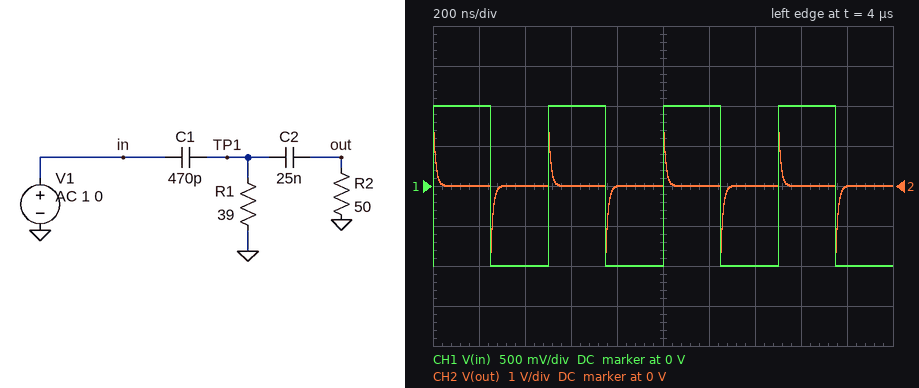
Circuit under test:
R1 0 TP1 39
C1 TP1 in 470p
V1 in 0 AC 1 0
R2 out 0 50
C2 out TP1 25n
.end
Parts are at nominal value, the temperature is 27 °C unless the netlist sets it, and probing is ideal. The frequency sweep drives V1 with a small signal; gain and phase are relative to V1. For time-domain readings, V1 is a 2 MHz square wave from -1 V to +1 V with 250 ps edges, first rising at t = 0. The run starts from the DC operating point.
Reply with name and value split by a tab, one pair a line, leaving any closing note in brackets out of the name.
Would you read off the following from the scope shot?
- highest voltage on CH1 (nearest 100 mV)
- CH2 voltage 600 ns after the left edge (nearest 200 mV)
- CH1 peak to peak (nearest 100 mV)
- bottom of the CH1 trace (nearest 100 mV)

highest voltage on CH1	1.0 V
CH2 voltage 600 ns after the left edge	0 V
CH1 peak to peak	2.0 V
bottom of the CH1 trace	-1.0 V
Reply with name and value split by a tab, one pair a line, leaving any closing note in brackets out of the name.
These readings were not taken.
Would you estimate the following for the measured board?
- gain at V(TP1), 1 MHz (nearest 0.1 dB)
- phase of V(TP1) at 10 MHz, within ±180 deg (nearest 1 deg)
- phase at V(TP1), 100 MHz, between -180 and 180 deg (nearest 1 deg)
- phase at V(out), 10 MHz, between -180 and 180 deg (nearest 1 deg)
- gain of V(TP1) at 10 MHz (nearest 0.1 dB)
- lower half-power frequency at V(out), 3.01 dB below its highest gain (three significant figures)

gain at V(TP1), 1 MHz	-23.8 dB
phase of V(TP1) at 10 MHz, within ±180 deg	57 deg
phase at V(TP1), 100 MHz, between -180 and 180 deg	9 deg
phase at V(out), 10 MHz, between -180 and 180 deg	58 deg
gain of V(TP1) at 10 MHz	-5.3 dB
lower half-power frequency at V(out), 3.01 dB below its highest gain	15.5 MHz
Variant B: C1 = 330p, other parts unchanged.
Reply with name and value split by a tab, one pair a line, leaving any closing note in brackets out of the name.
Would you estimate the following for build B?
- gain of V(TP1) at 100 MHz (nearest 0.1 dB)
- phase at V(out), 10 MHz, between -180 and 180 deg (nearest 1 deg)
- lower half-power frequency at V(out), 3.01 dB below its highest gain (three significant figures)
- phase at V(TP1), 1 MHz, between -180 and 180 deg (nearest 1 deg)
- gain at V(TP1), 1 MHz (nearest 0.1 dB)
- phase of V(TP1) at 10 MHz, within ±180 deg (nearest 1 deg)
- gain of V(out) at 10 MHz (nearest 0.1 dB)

gain of V(TP1) at 100 MHz	-0.2 dB
phase at V(out), 10 MHz, between -180 and 180 deg	66 deg
lower half-power frequency at V(out), 3.01 dB below its highest gain	22.1 MHz
phase at V(TP1), 1 MHz, between -180 and 180 deg	84 deg
gain at V(TP1), 1 MHz	-26.8 dB
phase of V(TP1) at 10 MHz, within ±180 deg	65 deg
gain of V(out) at 10 MHz	-7.7 dB
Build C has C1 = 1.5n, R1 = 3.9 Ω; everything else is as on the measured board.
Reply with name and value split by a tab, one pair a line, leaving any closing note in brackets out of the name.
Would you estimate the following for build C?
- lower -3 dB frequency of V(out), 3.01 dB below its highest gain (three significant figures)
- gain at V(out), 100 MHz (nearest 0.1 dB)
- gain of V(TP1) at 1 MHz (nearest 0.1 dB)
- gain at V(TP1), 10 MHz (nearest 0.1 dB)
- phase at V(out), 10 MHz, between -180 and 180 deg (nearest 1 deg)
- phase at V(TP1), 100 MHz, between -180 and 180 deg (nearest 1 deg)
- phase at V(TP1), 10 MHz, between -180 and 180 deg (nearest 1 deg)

lower -3 dB frequency of V(out), 3.01 dB below its highest gain	29.3 MHz
gain at V(out), 100 MHz	-0.4 dB
gain of V(TP1) at 1 MHz	-29.3 dB
gain at V(TP1), 10 MHz	-9.8 dB
phase at V(out), 10 MHz, between -180 and 180 deg	72 deg
phase at V(TP1), 100 MHz, between -180 and 180 deg	16 deg
phase at V(TP1), 10 MHz, between -180 and 180 deg	71 deg
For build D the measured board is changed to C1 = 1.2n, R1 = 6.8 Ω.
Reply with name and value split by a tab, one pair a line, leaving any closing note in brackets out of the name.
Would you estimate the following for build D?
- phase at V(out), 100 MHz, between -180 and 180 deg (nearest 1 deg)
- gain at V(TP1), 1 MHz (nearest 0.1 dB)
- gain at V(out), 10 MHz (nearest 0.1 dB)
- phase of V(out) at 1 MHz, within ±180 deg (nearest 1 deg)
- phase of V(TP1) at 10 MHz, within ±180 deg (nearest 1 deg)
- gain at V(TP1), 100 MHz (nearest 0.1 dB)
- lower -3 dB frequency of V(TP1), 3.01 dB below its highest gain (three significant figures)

phase at V(out), 100 MHz, between -180 and 180 deg	13 deg
gain at V(TP1), 1 MHz	-26.9 dB
gain at V(out), 10 MHz	-7.7 dB
phase of V(out) at 1 MHz, within ±180 deg	94 deg
phase of V(TP1) at 10 MHz, within ±180 deg	66 deg
gain at V(TP1), 100 MHz	-0.2 dB
lower -3 dB frequency of V(TP1), 3.01 dB below its highest gain	22.2 MHz
